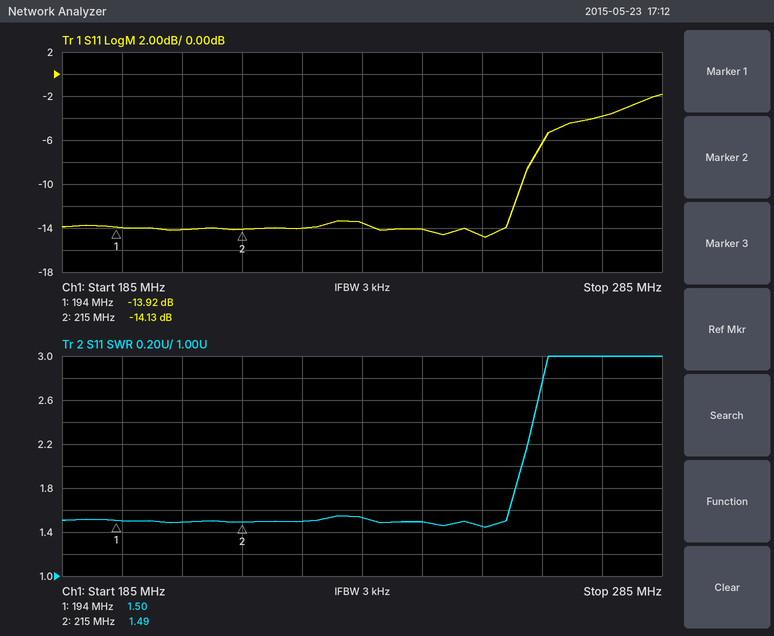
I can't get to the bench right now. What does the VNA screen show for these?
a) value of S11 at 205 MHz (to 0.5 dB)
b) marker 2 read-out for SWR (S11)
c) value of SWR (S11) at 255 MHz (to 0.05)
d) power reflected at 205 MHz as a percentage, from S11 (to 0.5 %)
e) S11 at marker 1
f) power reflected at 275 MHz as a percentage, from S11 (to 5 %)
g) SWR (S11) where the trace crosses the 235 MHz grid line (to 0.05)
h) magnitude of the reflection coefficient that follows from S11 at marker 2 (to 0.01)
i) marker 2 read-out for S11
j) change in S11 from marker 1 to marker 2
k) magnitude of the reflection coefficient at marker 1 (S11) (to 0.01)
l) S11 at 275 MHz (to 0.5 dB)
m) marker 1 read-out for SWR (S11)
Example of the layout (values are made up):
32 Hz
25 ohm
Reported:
-14.0 dB
1.49
1.45
4.0 %
-13.92 dB
40 %
1.55
0.20
-14.13 dB
-0.21 dB
0.20
-4.0 dB
1.50
